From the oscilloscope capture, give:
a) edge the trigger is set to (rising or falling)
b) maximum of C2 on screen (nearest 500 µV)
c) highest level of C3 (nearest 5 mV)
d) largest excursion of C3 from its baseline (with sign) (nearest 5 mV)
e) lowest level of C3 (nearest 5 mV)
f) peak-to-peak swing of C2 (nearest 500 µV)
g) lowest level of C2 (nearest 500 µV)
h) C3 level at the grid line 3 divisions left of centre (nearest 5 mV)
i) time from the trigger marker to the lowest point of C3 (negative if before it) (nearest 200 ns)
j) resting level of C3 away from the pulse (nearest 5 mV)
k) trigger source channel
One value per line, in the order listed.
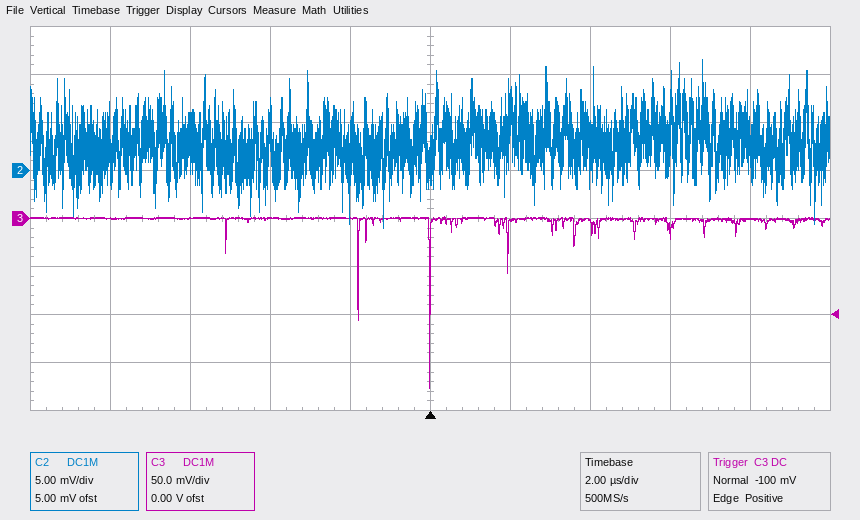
rising
11.5 mV
0 mV
-175 mV
-175 mV
17.5 mV
-6.0 mV
0 mV
0.0 µs
0 mV
C3
